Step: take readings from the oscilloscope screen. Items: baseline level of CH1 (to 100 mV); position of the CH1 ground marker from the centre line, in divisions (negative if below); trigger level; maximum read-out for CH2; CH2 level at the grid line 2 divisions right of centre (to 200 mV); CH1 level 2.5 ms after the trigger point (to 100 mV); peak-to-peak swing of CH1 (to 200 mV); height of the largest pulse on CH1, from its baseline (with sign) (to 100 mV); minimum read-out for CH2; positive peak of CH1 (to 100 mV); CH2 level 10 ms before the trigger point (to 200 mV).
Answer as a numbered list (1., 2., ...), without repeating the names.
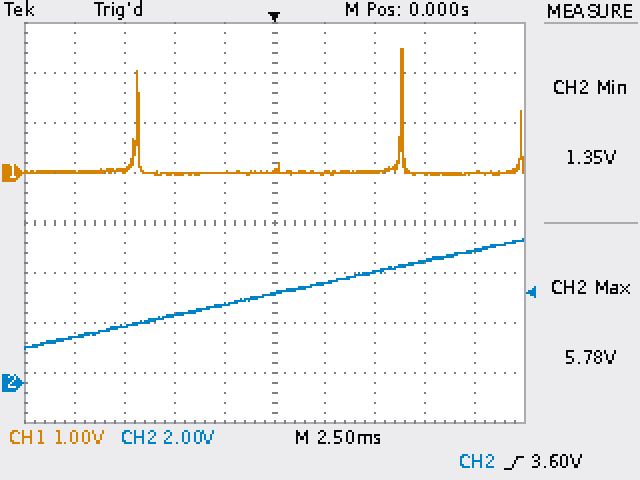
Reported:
1. 0.0 V
2. +1.0 div
3. 3.60 V
4. 5.78 V
5. 4.4 V
6. 0.0 V
7. 2.6 V
8. +2.5 V
9. 1.35 V
10. 2.5 V
11. 1.8 V
